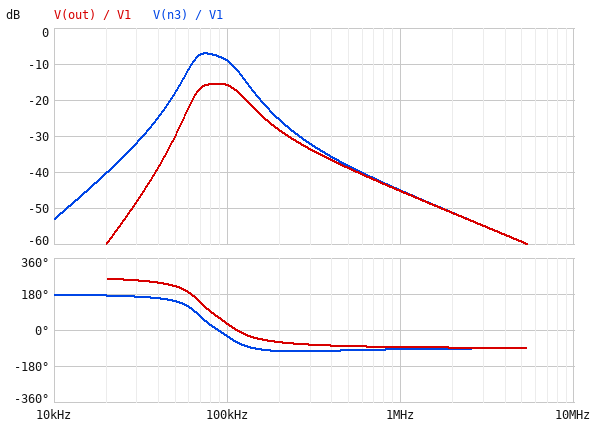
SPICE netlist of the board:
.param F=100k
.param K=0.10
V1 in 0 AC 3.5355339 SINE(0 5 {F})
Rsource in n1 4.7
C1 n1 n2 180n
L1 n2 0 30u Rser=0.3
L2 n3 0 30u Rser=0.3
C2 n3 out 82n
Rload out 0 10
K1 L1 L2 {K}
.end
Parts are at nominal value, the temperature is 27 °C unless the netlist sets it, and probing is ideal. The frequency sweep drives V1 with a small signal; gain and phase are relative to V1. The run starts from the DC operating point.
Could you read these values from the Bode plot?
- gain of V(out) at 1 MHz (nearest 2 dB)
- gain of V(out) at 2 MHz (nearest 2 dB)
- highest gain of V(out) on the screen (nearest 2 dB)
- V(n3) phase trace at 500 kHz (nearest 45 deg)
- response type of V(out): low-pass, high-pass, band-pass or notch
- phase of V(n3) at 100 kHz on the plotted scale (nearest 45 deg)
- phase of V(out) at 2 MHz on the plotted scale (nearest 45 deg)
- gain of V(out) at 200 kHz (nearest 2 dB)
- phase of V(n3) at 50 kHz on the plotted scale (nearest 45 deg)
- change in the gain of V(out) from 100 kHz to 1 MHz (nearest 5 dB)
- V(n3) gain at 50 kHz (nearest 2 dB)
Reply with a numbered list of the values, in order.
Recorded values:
1. -46 dB
2. -52 dB
3. -16 dB
4. -90 deg
5. band-pass
6. -45 deg
7. -90 deg
8. -28 dB
9. 135 deg
10. -30 dB
11. -18 dB
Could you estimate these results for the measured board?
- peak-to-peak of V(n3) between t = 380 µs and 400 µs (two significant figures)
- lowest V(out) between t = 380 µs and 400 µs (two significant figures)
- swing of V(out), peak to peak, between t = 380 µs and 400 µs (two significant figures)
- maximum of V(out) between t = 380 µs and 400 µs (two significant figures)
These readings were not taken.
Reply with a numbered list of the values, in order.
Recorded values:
1. 3.5 V
2. -800 mV
3. 1.6 V
4. 800 mV
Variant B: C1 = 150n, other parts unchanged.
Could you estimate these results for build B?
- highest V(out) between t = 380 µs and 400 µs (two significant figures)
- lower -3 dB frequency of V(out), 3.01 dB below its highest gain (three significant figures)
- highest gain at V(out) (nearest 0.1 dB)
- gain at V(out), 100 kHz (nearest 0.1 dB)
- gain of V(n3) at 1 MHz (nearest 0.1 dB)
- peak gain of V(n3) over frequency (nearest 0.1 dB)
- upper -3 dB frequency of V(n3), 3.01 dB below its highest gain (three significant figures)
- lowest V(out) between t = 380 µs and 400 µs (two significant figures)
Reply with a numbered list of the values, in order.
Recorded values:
1. 930 mV
2. 70.8 kHz
3. -13.8 dB
4. -14.6 dB
5. -45.1 dB
6. -5.6 dB
7. 104 kHz
8. -930 mV
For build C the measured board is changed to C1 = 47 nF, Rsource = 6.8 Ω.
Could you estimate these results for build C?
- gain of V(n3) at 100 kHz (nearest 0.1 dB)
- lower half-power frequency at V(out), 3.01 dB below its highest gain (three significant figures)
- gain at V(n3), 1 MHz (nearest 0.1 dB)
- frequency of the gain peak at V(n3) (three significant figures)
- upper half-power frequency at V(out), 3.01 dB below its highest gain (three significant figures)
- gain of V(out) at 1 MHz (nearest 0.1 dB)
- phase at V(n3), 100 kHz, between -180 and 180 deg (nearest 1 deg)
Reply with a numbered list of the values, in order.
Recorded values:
1. -12.5 dB
2. 112 kHz
3. -45.0 dB
4. 130 kHz
5. 151 kHz
6. -45.2 dB
7. 94 deg
